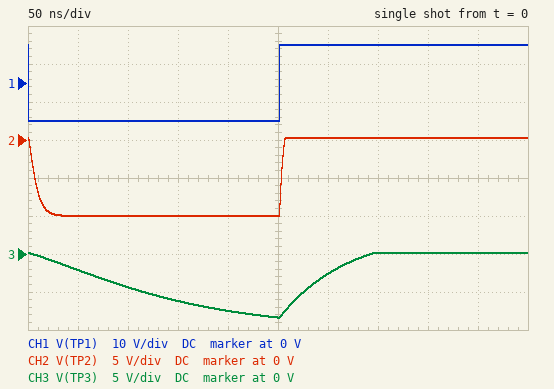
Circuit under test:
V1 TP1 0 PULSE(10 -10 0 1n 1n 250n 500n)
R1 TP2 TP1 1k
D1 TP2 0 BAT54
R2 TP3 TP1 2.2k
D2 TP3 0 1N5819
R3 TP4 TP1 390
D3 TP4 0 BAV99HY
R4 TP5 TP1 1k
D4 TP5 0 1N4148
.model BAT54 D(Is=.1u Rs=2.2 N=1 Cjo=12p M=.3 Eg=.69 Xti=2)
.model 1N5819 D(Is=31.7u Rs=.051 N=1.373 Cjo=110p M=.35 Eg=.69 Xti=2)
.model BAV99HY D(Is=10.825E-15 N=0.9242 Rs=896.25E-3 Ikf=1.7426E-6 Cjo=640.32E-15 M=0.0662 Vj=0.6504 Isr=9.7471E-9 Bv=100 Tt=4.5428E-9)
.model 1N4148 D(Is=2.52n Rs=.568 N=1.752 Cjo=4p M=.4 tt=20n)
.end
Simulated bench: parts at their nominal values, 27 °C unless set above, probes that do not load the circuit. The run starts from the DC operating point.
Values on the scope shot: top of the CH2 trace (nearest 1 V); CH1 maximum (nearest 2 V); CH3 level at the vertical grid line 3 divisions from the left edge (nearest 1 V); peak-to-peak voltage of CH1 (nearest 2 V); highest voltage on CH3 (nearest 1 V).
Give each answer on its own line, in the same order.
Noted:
0 V
10 V
-6 V
20 V
0 V
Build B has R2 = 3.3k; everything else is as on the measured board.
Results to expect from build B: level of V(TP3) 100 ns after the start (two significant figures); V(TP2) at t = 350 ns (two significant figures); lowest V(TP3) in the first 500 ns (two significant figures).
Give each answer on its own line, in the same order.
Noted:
-2.9 V
320 mV
-6.7 V
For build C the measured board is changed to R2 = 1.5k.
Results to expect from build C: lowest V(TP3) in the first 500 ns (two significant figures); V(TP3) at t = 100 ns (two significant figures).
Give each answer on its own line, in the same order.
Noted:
-9.4 V
-6.1 V
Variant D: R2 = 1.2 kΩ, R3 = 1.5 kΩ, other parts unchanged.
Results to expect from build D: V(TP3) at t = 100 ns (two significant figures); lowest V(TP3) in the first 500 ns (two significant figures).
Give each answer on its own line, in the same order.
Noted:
-7.1 V
-9.7 V
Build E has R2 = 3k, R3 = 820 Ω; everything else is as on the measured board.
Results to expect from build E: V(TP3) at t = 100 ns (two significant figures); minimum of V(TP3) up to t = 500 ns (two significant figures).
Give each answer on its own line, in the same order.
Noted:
-3.2 V
-7.1 V
